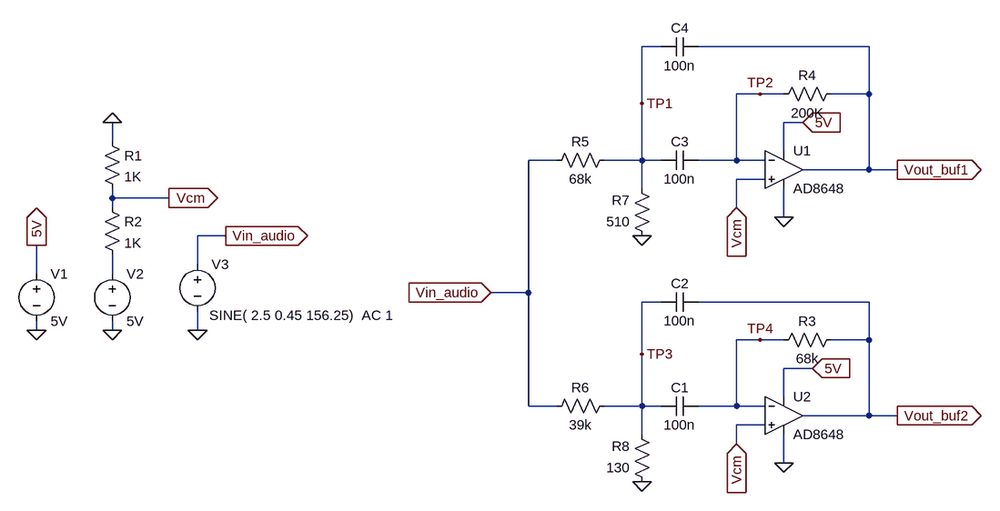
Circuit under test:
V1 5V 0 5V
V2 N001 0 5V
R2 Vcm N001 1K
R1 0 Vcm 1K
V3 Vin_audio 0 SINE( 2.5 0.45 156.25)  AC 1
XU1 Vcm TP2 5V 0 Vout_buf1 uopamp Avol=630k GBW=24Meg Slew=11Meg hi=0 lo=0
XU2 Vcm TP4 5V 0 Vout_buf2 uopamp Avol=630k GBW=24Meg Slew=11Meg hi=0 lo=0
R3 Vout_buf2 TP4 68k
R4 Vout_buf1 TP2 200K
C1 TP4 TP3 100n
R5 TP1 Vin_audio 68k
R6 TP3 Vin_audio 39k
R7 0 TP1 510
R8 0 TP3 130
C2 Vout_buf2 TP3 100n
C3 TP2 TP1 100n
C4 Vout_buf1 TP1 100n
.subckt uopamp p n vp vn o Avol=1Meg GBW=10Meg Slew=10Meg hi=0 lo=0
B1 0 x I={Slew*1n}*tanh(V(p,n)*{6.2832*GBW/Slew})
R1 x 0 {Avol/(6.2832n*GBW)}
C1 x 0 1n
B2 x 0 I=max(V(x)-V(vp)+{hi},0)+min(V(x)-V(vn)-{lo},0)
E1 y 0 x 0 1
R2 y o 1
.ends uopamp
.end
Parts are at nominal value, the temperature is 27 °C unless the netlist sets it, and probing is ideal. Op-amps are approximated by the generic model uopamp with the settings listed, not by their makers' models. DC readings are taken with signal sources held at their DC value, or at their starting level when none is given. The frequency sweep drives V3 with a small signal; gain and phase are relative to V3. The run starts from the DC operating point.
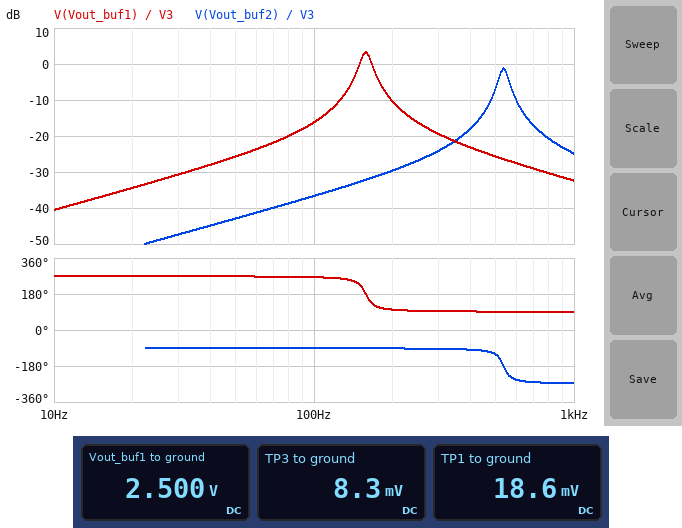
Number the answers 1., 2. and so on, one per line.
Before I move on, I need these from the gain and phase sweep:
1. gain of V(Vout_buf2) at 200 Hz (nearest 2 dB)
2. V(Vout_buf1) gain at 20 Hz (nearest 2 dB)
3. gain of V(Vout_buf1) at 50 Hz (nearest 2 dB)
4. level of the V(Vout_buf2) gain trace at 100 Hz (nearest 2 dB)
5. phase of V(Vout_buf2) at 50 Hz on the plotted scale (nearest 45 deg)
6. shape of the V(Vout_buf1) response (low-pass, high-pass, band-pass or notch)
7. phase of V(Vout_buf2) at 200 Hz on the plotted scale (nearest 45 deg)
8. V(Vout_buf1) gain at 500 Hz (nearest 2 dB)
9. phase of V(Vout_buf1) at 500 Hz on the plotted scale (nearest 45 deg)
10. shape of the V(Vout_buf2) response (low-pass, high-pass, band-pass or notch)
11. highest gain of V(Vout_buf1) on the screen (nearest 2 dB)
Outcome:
1. -30 dB
2. -34 dB
3. -26 dB
4. -36 dB
5. -90 deg
6. band-pass
7. -90 deg
8. -26 dB
9. 90 deg
10. band-pass
11. 4 dB
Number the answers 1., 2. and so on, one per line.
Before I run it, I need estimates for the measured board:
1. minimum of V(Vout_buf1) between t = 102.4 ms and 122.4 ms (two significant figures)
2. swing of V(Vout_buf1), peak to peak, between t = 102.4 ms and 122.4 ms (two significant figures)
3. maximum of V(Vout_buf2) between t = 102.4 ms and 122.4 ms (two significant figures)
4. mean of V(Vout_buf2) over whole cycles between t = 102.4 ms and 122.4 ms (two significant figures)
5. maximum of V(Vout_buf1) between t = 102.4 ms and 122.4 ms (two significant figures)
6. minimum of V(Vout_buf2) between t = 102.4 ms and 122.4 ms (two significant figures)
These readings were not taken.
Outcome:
1. 1.9 V
2. 1.3 V
3. 2.5 V
4. 2.5 V
5. 3.1 V
6. 2.5 V
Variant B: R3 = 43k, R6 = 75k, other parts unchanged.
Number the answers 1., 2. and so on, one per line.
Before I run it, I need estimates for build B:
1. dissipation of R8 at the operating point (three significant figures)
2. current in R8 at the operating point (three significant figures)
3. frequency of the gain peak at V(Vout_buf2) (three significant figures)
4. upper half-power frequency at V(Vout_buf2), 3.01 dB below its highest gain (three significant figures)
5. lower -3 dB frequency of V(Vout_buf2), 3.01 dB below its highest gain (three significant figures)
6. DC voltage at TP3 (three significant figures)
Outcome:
1. 144 nW
2. 33.3 µA
3. 674 Hz
4. 712 Hz
5. 638 Hz
6. 4.33 mV
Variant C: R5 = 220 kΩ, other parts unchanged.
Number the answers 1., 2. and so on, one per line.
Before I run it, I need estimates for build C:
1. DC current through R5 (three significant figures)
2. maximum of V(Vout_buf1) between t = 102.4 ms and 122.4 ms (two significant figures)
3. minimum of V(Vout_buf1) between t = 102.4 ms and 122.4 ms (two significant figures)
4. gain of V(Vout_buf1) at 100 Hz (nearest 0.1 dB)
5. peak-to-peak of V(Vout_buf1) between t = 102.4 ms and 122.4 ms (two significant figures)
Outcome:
1. 11.3 µA
2. 2.7 V
3. 2.3 V
4. -26.3 dB
5. 400 mV
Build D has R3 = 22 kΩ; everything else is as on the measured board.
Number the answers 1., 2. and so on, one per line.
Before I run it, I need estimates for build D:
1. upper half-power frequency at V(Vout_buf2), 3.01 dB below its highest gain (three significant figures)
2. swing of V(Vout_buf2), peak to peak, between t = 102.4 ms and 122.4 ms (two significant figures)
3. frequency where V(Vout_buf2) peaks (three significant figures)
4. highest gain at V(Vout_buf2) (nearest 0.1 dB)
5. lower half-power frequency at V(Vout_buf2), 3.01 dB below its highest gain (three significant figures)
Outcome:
1. 1.02 kHz
2. 6.6 mV
3. 942 Hz
4. -11.0 dB
5. 873 Hz
